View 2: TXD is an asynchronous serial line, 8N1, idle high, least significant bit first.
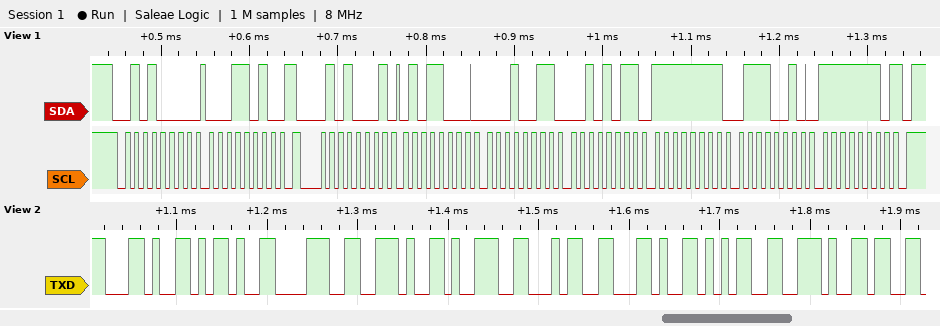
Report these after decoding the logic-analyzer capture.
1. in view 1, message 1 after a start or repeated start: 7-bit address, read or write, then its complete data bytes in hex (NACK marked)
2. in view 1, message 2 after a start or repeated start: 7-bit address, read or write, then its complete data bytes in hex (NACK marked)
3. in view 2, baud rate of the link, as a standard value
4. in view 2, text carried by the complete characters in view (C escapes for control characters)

0x28 write: 1A
0x28 read: 58 13 2B FF 72 FE NACK
115200 baud
",-8.94,5."
